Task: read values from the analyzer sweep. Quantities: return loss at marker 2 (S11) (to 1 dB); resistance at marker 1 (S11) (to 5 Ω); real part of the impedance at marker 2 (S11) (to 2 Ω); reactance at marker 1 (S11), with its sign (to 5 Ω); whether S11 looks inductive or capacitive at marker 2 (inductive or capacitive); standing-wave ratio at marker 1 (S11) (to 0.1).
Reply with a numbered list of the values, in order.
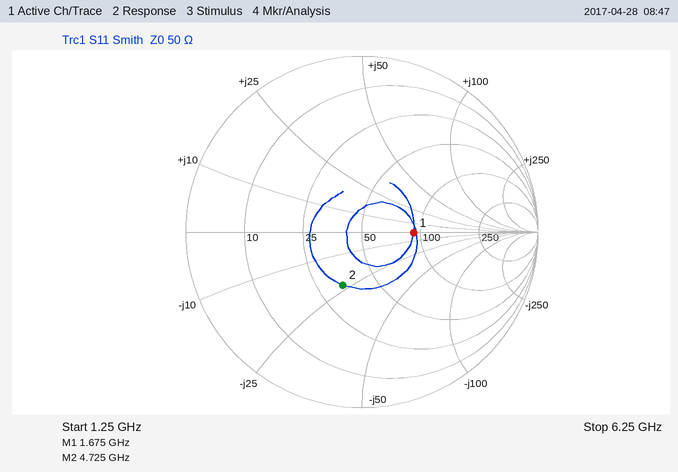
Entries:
1. 10 dB
2. 90 Ω
3. 34 Ω
4. 0 Ω
5. capacitive
6. 1.8
